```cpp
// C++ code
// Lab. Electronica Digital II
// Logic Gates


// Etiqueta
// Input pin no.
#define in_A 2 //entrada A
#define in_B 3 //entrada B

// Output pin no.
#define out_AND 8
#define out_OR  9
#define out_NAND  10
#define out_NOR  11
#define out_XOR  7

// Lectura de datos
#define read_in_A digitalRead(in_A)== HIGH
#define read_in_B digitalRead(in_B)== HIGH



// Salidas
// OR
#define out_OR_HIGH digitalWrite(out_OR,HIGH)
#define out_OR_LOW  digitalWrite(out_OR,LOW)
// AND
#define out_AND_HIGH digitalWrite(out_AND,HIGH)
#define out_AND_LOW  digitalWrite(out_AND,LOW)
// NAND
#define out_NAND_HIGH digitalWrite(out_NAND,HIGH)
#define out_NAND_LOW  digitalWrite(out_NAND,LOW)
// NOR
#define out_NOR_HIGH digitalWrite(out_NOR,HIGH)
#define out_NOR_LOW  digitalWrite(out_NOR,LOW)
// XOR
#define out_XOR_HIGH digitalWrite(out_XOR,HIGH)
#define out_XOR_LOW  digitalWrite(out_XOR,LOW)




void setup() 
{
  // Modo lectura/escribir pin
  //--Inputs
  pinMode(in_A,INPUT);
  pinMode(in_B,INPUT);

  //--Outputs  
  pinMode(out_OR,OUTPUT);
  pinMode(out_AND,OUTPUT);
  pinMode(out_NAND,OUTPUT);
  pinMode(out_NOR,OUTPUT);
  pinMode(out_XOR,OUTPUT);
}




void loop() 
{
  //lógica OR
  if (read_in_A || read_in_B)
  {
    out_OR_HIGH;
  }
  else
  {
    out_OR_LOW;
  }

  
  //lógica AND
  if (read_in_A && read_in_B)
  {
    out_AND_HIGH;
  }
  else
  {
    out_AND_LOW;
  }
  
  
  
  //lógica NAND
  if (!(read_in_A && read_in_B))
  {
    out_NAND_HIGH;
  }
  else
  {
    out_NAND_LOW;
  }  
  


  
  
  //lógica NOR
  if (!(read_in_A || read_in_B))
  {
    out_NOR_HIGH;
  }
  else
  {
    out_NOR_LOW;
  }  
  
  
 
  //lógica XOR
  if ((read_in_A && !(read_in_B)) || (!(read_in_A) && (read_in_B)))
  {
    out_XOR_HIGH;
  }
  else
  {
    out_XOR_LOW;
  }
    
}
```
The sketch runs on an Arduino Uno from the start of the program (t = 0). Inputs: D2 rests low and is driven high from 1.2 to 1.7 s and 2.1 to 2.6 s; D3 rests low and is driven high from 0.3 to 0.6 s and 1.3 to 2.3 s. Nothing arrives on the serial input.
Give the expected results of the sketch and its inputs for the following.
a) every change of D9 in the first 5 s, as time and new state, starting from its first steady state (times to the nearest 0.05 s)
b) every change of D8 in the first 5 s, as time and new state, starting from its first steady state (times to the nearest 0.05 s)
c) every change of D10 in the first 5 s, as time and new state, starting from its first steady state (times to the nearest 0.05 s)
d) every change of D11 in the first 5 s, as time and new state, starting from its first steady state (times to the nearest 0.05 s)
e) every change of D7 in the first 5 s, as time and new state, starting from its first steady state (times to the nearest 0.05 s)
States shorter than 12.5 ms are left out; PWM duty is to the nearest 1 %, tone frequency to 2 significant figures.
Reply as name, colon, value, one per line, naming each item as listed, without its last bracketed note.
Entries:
every change of D9 in the first 5 s, as time and new state, starting from its first steady state: 0 s low; 0.3 s high; 0.6 s low; 1.2 s high; 2.6 s low
every change of D8 in the first 5 s, as time and new state, starting from its first steady state: 0 s low; 1.3 s high; 1.7 s low; 2.1 s high; 2.3 s low
every change of D10 in the first 5 s, as time and new state, starting from its first steady state: 0 s high; 1.3 s low; 1.7 s high; 2.1 s low; 2.3 s high
every change of D11 in the first 5 s, as time and new state, starting from its first steady state: 0 s high; 0.3 s low; 0.6 s high; 1.2 s low; 2.6 s high
every change of D7 in the first 5 s, as time and new state, starting from its first steady state: 0 s low; 0.3 s high; 0.6 s low; 1.2 s high; 1.3 s low; 1.7 s high; 2.1 s low; 2.3 s high; 2.6 s low
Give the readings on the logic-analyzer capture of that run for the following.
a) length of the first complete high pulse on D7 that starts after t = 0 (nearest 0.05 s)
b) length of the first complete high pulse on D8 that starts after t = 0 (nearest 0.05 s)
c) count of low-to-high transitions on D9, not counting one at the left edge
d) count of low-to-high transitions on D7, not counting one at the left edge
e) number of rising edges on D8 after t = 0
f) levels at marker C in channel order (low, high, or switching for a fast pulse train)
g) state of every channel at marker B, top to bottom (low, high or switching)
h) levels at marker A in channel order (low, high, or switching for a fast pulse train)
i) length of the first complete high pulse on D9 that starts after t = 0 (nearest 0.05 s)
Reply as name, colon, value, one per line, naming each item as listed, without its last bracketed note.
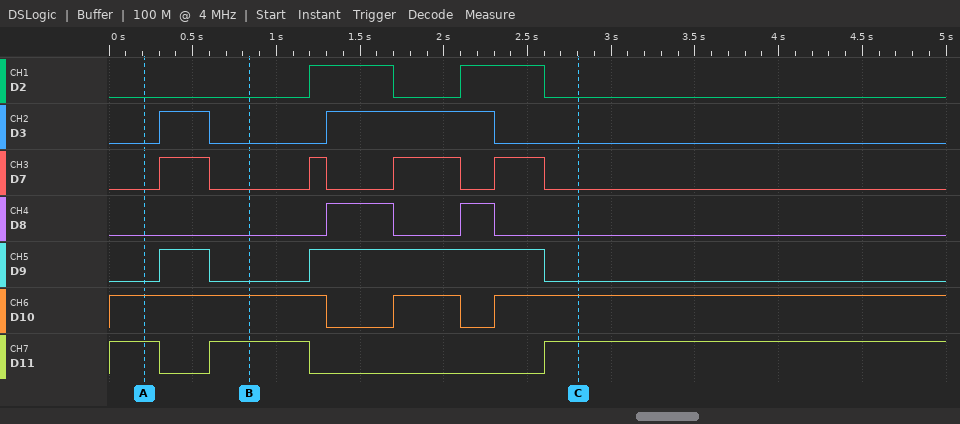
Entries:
length of the first complete high pulse on D7 that starts after t = 0: 0.30 s
length of the first complete high pulse on D8 that starts after t = 0: 0.40 s
count of low-to-high transitions on D9, not counting one at the left edge: 2
count of low-to-high transitions on D7, not counting one at the left edge: 4
number of rising edges on D8 after t = 0: 2
levels at marker C in channel order: D2 low, D3 low, D7 low, D8 low, D9 low, D10 high, D11 high
state of every channel at marker B, top to bottom: D2 low, D3 low, D7 low, D8 low, D9 low, D10 high, D11 high
levels at marker A in channel order: D2 low, D3 low, D7 low, D8 low, D9 low, D10 high, D11 high
length of the first complete high pulse on D9 that starts after t = 0: 0.30 s
